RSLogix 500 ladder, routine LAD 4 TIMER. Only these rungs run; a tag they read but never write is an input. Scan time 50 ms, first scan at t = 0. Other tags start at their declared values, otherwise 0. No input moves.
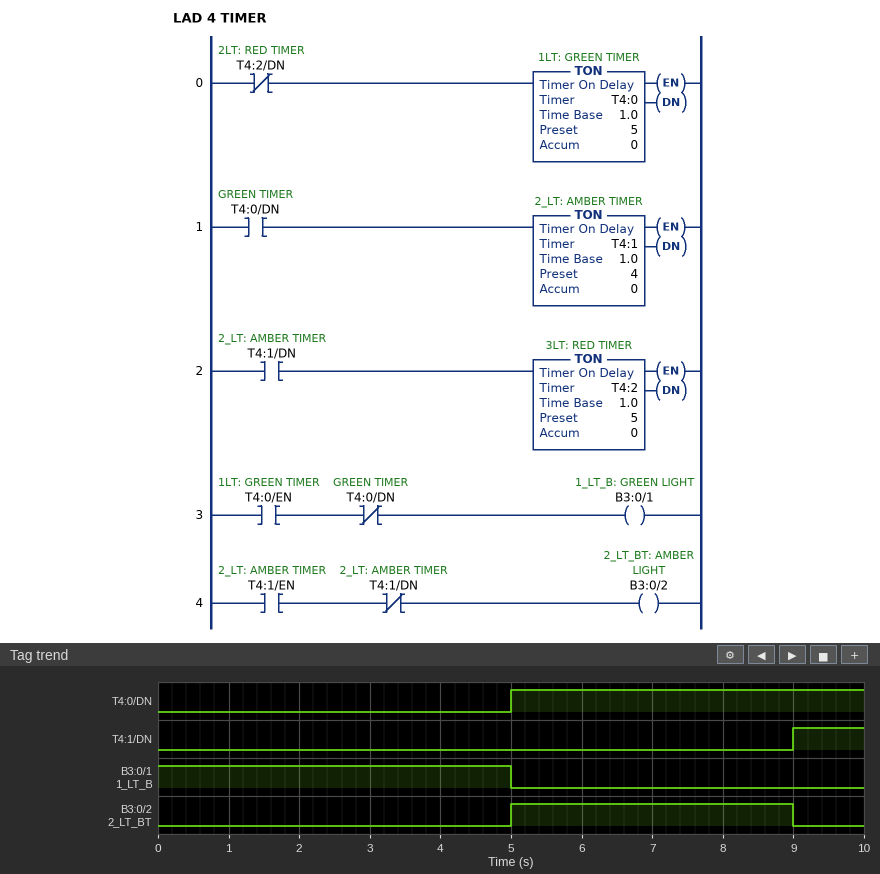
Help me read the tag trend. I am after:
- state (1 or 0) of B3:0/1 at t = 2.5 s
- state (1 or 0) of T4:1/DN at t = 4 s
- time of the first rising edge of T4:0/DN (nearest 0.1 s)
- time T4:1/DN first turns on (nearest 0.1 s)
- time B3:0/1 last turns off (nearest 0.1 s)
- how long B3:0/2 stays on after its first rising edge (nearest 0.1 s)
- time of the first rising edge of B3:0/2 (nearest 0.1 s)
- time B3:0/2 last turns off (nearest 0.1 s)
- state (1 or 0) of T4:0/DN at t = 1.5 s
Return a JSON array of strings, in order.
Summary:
["1", "0", "5.0 s", "9.0 s", "5.0 s", "4.0 s", "5.0 s", "9.0 s", "0"]
